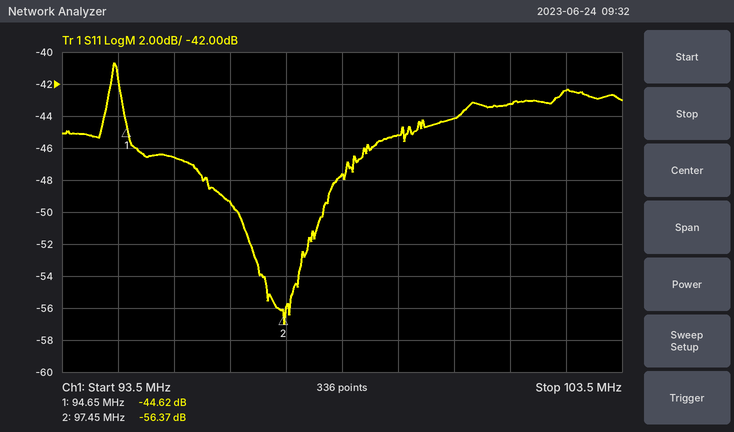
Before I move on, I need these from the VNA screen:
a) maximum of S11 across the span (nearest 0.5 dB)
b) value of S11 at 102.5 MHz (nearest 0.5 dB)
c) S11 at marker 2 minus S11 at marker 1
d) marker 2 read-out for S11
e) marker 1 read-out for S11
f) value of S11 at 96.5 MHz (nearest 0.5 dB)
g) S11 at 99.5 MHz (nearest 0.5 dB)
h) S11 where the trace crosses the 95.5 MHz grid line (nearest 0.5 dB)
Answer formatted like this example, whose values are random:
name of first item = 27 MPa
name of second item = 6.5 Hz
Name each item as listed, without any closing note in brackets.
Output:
maximum of S11 across the span = -40.5 dB
value of S11 at 102.5 MHz = -42.5 dB
S11 at marker 2 minus S11 at marker 1 = -11.75 dB
marker 2 read-out for S11 = -56.37 dB
marker 1 read-out for S11 = -44.62 dB
value of S11 at 96.5 MHz = -49.5 dB
S11 at 99.5 MHz = -45.0 dB
S11 where the trace crosses the 95.5 MHz grid line = -46.5 dB
